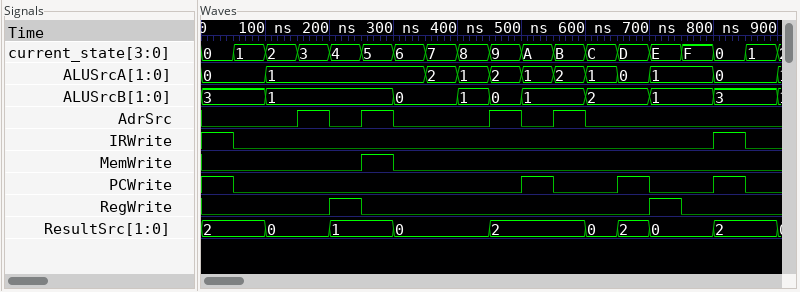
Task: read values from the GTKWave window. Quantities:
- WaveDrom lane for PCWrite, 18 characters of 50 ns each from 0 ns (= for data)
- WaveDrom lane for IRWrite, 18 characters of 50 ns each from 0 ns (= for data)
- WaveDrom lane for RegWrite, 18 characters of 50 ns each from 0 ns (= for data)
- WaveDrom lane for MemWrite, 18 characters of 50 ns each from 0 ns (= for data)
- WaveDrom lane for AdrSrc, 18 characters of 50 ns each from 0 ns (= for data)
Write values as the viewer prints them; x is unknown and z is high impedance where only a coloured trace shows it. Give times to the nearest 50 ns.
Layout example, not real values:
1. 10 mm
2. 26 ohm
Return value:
1. {name: 'PCWrite', wave: '10........10.10.10'}
2. {name: 'IRWrite', wave: '10..............10'}
3. {name: 'RegWrite', wave: '0...10........10..'}
4. {name: 'MemWrite', wave: '0....10...........'}
5. {name: 'AdrSrc', wave: '0..1010..1010.....'}
